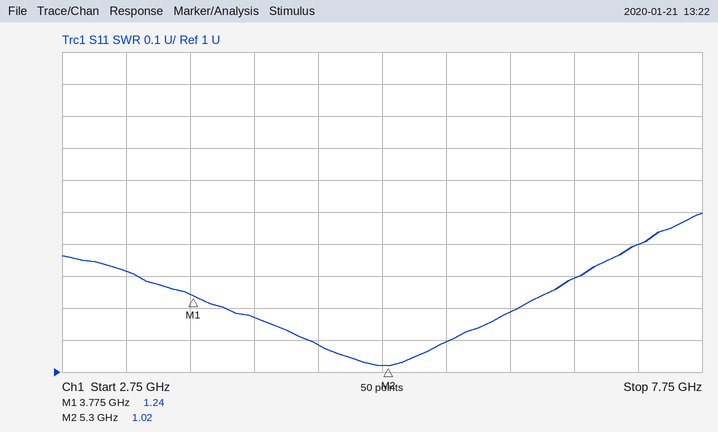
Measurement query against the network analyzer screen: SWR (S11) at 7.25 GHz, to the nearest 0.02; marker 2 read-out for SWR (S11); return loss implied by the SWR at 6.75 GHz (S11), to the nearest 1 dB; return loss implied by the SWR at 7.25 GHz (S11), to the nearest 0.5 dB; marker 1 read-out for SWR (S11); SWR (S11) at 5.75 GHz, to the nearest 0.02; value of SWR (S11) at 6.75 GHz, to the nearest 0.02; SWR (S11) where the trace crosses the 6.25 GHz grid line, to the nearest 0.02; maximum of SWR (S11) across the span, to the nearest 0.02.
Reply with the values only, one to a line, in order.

1.40
1.02
18 dB
15.5 dB
1.24
1.10
1.30
1.18
1.50
